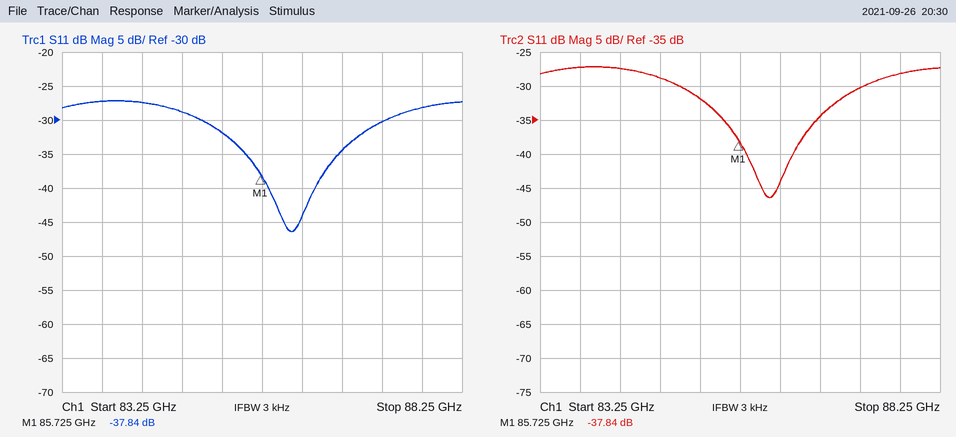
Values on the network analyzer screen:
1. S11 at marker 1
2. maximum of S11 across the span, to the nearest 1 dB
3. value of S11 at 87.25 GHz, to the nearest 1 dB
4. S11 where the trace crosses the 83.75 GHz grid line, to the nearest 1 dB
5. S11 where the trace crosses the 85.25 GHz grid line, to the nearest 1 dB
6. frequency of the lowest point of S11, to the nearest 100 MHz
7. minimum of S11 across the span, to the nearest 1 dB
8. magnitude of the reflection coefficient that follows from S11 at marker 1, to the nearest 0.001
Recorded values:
-37.84 dB
-27 dB
-30 dB
-27 dB
-32 dB
86.1 GHz
-46 dB
0.013
